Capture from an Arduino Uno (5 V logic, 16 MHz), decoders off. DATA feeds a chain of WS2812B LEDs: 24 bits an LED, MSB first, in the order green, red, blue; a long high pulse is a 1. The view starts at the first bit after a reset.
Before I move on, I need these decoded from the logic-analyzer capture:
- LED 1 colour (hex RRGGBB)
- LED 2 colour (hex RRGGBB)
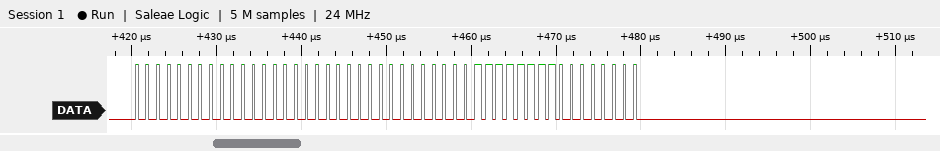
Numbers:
#000000
#FF0000
